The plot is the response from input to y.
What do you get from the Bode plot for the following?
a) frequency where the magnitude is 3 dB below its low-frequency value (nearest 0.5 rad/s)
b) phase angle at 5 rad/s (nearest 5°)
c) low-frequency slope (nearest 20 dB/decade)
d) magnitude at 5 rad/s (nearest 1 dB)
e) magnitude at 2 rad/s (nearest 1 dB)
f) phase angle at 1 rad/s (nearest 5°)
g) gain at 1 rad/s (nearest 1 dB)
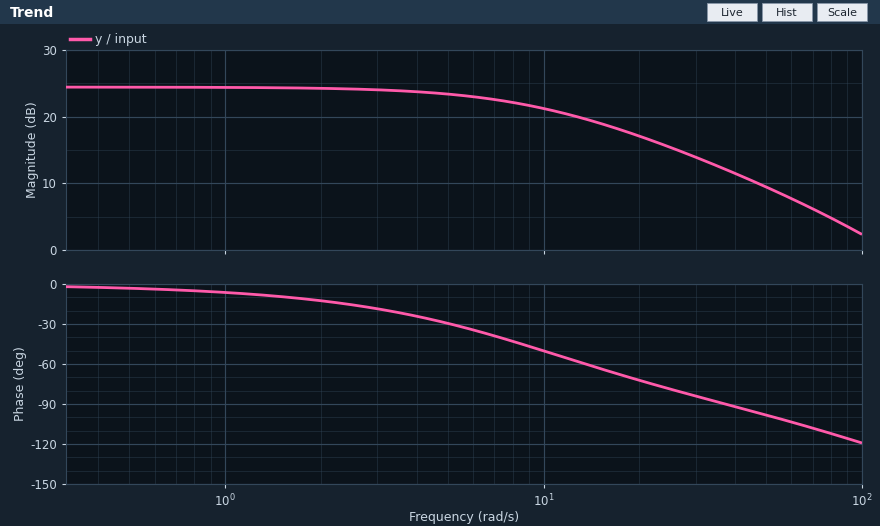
9.5 rad/s
-30°
0 dB/decade
23 dB
24 dB
-5°
24 dB
